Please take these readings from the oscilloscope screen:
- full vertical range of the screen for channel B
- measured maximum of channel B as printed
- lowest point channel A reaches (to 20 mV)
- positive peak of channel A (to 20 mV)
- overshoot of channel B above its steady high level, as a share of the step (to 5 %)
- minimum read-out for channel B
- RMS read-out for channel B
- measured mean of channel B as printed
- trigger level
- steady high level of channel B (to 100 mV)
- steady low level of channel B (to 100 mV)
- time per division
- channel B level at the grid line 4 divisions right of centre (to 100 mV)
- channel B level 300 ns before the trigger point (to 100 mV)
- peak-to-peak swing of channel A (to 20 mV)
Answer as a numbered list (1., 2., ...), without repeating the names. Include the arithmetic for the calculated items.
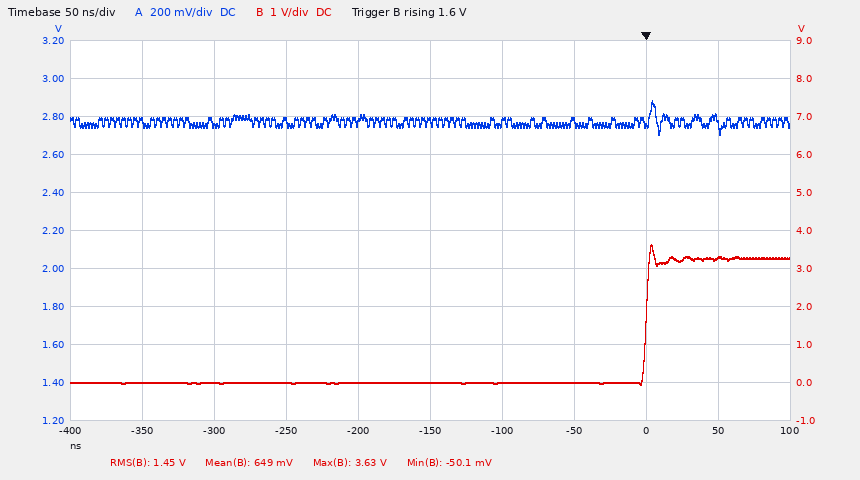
1. 10 V
2. 3.63 V
3. 2.70 V
4. 2.88 V
5. 10 %
6. -50.1 mV
7. 1.45 V
8. 649 mV
9. 1.6 V
10. 3.3 V
11. 0.0 V
12. 50 ns
13. 3.3 V
14. 0.0 V
15. 2.88 V − (2.70 V) = 180 mV
